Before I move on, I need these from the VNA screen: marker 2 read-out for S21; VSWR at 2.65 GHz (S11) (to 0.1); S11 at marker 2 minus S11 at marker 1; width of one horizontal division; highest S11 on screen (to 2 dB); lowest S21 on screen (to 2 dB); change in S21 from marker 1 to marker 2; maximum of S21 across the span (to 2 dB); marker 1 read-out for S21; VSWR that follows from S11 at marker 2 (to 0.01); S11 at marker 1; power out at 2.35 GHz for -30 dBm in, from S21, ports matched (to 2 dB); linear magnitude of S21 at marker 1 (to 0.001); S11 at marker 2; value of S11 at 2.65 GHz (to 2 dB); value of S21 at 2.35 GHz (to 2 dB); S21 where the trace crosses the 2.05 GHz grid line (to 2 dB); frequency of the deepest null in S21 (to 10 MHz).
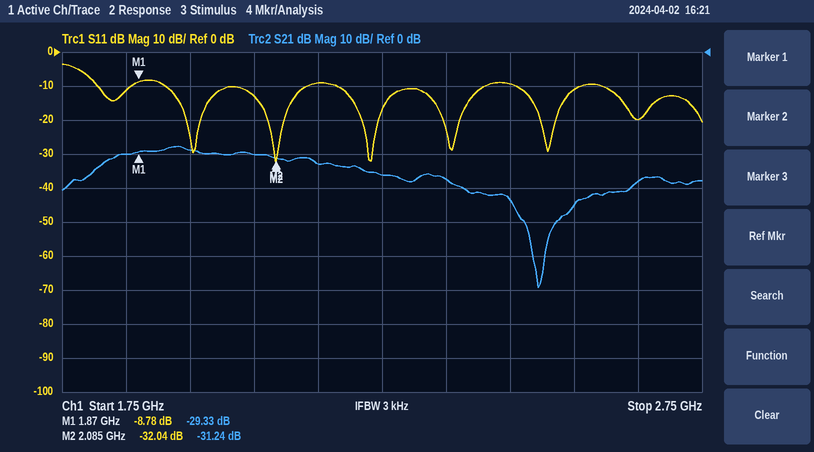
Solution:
-31.24 dB
1.2
-23.26 dB
100 MHz
-4 dB
-70 dB
-1.91 dB
-28 dB
-29.33 dB
1.05
-8.78 dB
-68 dBm
0.034
-32.04 dB
-20 dB
-38 dB
-30 dB
2.49 GHz
